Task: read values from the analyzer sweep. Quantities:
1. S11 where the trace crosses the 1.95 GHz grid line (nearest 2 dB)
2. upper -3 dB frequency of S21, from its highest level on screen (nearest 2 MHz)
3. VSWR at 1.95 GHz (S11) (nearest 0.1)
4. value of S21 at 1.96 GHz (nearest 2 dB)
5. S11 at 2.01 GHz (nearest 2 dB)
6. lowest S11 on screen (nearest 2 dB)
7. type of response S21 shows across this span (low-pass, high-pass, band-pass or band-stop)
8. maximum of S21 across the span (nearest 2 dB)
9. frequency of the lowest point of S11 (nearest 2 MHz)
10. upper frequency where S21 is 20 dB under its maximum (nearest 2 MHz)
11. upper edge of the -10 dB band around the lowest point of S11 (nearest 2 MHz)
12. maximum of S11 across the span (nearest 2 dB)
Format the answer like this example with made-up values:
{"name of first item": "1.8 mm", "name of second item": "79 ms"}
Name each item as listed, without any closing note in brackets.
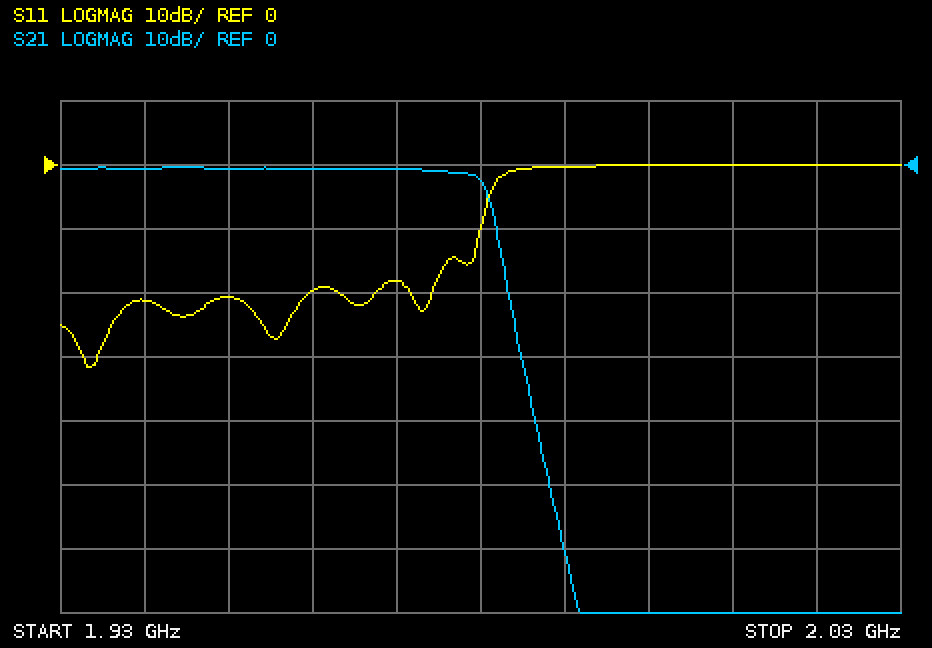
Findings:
{"S11 where the trace crosses the 1.95 GHz grid line": "-20 dB", "upper -3 dB frequency of S21, from its highest level on screen": "1.980 GHz", "VSWR at 1.95 GHz (S11)": "1.2", "value of S21 at 1.96 GHz": "0 dB", "S11 at 2.01 GHz": "0 dB", "lowest S11 on screen": "-32 dB", "type of response S21 shows across this span": "low-pass", "maximum of S21 across the span": "0 dB", "frequency of the lowest point of S11": "1.934 GHz", "upper frequency where S21 is 20 dB under its maximum": "1.984 GHz", "upper edge of the -10 dB band around the lowest point of S11": "1.980 GHz", "maximum of S11 across the span": "0 dB"}
